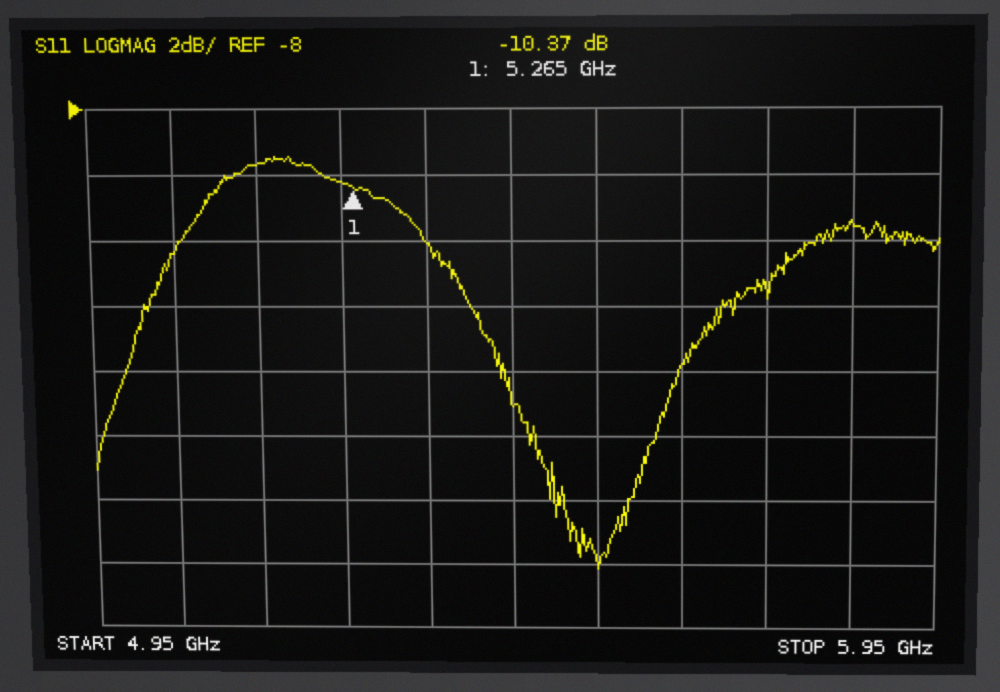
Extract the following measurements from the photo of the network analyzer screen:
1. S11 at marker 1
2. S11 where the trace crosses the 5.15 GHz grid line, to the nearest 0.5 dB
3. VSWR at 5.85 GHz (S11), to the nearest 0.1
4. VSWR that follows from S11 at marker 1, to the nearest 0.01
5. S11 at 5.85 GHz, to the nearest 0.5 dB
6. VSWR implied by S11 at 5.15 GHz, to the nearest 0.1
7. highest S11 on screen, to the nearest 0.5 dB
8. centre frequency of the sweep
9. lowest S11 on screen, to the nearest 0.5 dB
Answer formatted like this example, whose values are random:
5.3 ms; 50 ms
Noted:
-10.37 dB; -9.5 dB; 1.7; 1.87; -11.5 dB; 2.0; -9.5 dB; 5.45 GHz; -22.0 dB
